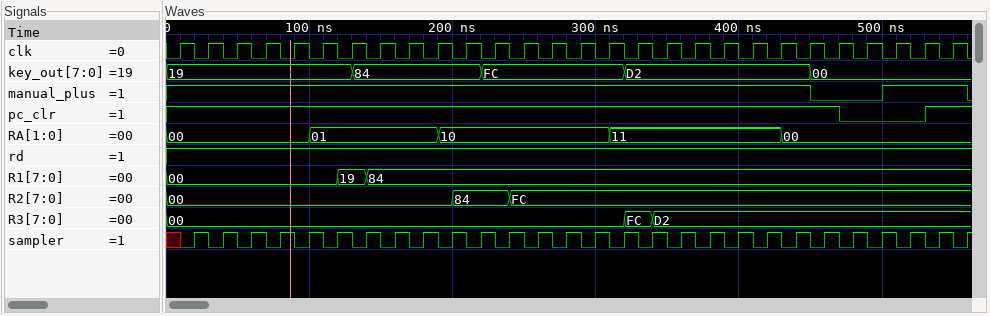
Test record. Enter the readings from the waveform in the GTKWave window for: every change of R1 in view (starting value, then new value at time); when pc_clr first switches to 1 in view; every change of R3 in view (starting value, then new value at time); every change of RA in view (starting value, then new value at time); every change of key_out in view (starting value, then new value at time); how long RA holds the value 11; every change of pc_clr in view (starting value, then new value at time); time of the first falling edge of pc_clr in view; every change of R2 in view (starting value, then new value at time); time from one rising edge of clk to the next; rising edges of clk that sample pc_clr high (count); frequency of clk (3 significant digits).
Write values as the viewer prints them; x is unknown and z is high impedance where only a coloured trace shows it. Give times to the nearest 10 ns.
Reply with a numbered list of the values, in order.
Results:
1. 00, 19 at 120 ns, 84 at 140 ns
2. 530 ns
3. 00, FC at 320 ns, D2 at 340 ns
4. 00, 01 at 100 ns, 10 at 190 ns, 11 at 310 ns, 00 at 430 ns
5. 19, 84 at 130 ns, FC at 220 ns, D2 at 320 ns, 00 at 450 ns
6. 120 ns
7. 1, 0 at 470 ns, 1 at 530 ns
8. 470 ns
9. 00, 84 at 200 ns, FC at 240 ns
10. 20 ns
11. 25
12. 50.0 MHz
